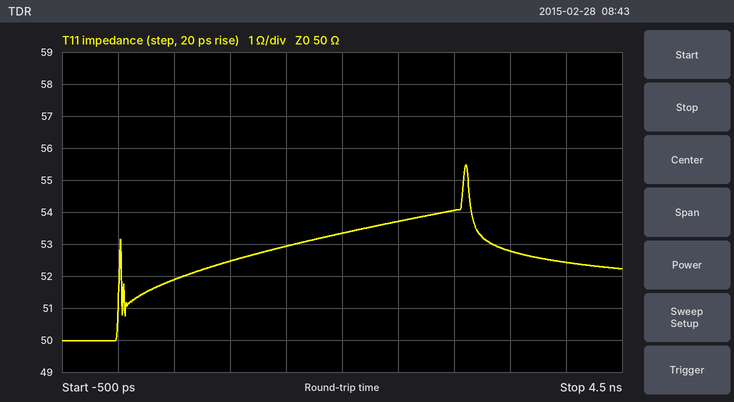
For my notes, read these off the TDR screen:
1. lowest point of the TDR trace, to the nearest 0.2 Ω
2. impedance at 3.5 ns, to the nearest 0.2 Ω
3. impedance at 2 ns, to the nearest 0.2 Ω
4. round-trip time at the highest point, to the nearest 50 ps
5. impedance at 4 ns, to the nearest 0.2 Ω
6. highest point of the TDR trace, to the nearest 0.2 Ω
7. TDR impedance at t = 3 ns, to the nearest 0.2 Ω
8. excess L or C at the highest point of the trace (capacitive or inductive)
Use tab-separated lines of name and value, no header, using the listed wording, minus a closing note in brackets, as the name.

lowest point of the TDR trace, to the nearest 0.2 Ω	50.0 Ω
impedance at 3.5 ns, to the nearest 0.2 Ω	52.8 Ω
impedance at 2 ns, to the nearest 0.2 Ω	53.4 Ω
round-trip time at the highest point, to the nearest 50 ps	3.10 ns
impedance at 4 ns, to the nearest 0.2 Ω	52.4 Ω
highest point of the TDR trace, to the nearest 0.2 Ω	55.4 Ω
TDR impedance at t = 3 ns, to the nearest 0.2 Ω	54.0 Ω
excess L or C at the highest point of the trace	inductive
